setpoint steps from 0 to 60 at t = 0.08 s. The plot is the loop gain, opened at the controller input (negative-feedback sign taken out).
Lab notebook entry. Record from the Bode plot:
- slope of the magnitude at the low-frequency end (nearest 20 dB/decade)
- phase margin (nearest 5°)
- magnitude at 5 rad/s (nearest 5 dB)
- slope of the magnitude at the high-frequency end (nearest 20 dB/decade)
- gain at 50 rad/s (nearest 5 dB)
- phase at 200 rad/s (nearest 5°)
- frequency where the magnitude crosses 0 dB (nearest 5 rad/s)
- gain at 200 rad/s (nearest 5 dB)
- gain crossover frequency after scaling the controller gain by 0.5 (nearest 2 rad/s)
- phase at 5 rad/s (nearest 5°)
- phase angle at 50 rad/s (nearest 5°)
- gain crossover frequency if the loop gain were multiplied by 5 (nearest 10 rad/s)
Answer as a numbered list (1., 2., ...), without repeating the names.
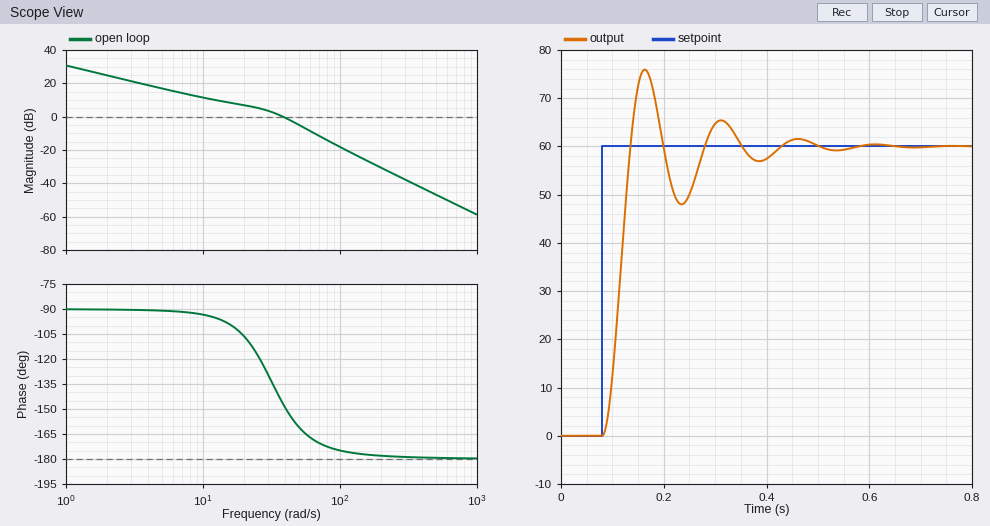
1. -20 dB/decade
2. 35°
3. 15 dB
4. -40 dB/decade
5. -5 dB
6. -180°
7. 40 rad/s
8. -30 dB
9. 22 rad/s
10. -90°
11. -160°
12. 80 rad/s
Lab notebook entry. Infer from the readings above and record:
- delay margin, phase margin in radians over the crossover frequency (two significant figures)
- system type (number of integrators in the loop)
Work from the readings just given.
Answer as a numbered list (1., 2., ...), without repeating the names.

1. 0.015 s
2. 1
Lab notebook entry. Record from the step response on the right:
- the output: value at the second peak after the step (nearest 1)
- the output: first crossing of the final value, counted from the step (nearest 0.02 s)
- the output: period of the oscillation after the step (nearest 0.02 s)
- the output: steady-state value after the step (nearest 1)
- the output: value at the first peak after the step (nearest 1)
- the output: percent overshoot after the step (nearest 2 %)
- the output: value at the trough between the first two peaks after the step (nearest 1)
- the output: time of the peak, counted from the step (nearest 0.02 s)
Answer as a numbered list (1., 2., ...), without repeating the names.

1. 65
2. 0.06 s
3. 0.14 s
4. 60
5. 76
6. 26 %
7. 48
8. 0.08 s
